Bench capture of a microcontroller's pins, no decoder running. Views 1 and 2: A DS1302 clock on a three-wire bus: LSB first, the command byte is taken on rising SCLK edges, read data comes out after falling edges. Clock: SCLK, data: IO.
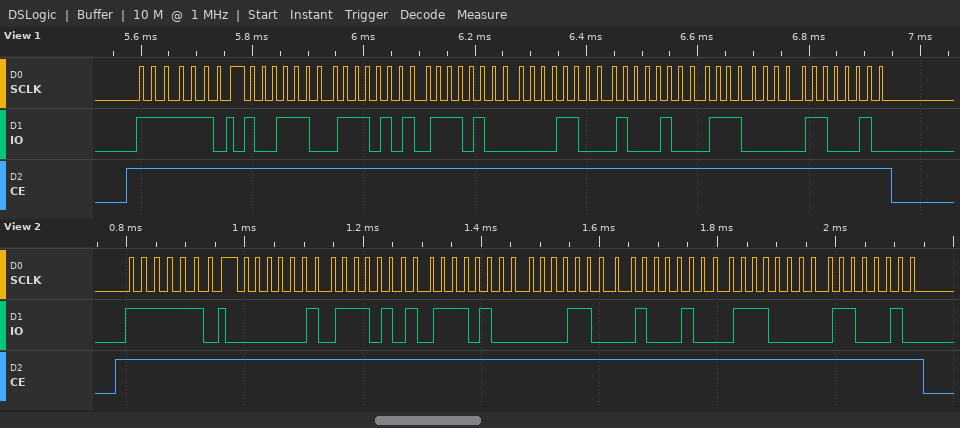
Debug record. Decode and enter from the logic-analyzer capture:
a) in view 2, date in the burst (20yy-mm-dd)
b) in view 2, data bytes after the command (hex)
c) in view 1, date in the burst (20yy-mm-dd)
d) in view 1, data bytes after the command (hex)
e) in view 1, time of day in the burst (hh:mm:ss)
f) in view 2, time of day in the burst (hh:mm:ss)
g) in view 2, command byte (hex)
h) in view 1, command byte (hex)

2023-11-18
40 57 17 18 11 07 23
2023-11-18
39 57 17 18 11 07 23
17:57:39
17:57:40
0xBF
0xBF
